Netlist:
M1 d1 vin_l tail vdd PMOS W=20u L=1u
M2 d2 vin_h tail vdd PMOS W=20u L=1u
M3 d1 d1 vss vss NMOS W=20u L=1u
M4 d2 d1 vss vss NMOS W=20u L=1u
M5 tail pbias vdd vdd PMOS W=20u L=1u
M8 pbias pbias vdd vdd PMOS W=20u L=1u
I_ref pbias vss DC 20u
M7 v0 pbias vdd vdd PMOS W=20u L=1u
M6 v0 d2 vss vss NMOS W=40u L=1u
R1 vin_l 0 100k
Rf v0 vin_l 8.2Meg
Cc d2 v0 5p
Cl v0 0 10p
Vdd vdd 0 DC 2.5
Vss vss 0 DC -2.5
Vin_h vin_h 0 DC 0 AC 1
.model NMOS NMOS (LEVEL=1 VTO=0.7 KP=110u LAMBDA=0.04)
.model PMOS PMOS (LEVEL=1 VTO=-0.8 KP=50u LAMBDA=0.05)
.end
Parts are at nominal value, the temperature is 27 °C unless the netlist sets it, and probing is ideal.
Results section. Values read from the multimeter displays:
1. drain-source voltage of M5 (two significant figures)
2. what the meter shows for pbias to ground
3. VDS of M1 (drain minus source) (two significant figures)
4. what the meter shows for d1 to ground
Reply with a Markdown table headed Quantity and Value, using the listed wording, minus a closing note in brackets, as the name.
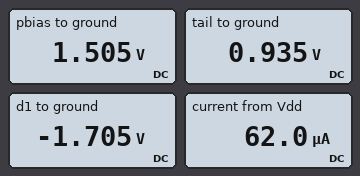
| Quantity | Value |
|---|---|
| drain-source voltage of M5 | -1.6 V |
| what the meter shows for pbias to ground | 1.505 V |
| VDS of M1 (drain minus source) | -2.6 V |
| what the meter shows for d1 to ground | -1.705 V |
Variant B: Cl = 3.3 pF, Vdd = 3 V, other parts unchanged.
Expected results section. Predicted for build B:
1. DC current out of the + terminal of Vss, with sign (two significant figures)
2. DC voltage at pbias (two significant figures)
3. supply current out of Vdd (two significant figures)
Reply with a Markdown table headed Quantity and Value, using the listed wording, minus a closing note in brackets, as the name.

| Quantity | Value |
|---|---|
| DC current out of the + terminal of Vss, with sign | -63 µA |
| DC voltage at pbias | 2.0 V |
| supply current out of Vdd | 63 µA |
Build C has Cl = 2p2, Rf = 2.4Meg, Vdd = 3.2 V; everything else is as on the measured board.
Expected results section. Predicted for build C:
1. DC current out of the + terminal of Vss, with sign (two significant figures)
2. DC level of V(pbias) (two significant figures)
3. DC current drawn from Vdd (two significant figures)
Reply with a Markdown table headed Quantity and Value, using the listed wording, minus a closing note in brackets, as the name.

| Quantity | Value |
|---|---|
| DC current out of the + terminal of Vss, with sign | -63 µA |
| DC level of V(pbias) | 2.2 V |
| DC current drawn from Vdd | 63 µA |
